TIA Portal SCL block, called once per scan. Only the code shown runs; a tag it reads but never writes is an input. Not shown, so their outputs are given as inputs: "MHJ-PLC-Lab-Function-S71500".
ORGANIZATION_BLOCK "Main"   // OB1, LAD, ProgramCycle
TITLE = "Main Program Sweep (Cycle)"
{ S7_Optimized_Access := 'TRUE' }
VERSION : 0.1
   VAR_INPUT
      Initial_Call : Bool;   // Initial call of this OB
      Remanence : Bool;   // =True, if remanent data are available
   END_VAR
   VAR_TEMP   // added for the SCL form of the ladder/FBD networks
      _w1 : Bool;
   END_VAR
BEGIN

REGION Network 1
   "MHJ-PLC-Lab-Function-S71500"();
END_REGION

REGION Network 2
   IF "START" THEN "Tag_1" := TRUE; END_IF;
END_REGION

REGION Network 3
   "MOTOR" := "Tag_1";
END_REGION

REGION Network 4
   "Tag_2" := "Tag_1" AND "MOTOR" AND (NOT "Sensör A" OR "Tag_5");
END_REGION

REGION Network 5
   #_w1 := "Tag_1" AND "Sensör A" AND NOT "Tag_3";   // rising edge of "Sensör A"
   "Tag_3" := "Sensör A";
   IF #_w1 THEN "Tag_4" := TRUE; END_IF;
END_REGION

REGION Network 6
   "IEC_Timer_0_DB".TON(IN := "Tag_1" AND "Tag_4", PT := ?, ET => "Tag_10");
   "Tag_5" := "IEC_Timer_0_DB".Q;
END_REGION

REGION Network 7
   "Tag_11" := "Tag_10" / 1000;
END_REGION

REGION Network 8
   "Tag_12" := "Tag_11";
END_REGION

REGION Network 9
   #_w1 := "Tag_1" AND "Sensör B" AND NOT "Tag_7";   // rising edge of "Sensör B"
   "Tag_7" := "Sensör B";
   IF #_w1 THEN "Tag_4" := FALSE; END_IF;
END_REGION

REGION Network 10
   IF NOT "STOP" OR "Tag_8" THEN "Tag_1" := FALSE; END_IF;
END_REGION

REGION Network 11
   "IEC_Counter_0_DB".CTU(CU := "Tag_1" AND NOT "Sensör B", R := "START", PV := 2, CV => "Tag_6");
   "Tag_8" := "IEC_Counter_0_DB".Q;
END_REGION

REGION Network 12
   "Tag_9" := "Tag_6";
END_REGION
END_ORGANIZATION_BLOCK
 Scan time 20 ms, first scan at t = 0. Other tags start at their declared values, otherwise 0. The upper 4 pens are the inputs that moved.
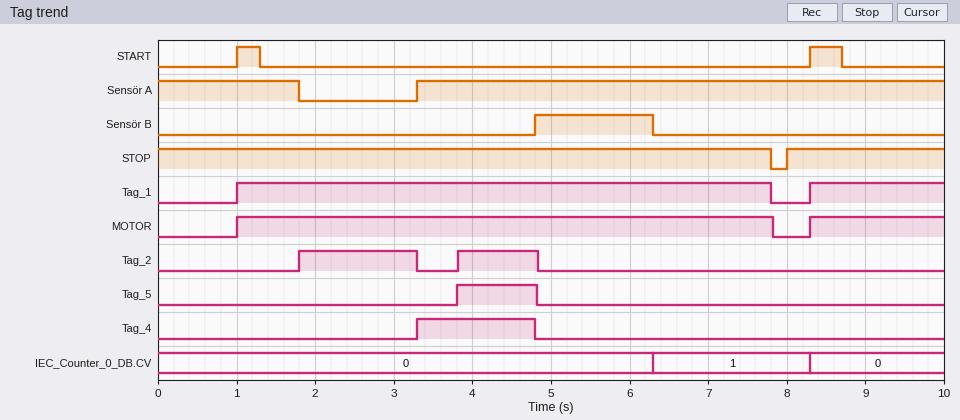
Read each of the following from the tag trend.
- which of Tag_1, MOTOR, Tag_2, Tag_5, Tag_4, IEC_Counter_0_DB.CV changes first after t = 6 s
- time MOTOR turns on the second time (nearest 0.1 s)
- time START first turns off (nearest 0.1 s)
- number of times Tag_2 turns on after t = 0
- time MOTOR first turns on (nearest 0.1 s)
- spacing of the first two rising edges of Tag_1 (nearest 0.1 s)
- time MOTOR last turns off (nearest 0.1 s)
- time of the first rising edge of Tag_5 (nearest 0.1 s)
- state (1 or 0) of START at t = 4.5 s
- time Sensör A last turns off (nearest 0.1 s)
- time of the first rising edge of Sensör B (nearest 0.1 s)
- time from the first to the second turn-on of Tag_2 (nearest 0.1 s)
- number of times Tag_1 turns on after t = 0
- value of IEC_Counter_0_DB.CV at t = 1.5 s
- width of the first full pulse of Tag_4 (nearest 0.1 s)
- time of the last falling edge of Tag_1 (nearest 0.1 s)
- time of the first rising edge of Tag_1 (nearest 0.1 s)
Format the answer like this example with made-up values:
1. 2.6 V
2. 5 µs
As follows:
1. IEC_Counter_0_DB.CV
2. 8.3 s
3. 1.3 s
4. 2
5. 1.0 s
6. 7.3 s
7. 7.8 s
8. 3.8 s
9. 0
10. 1.8 s
11. 4.8 s
12. 2.0 s
13. 2
14. 0
15. 1.5 s
16. 7.8 s
17. 1.0 s
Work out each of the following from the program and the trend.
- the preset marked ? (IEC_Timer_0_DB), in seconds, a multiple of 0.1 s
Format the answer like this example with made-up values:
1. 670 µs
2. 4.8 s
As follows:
1. 0.5 s
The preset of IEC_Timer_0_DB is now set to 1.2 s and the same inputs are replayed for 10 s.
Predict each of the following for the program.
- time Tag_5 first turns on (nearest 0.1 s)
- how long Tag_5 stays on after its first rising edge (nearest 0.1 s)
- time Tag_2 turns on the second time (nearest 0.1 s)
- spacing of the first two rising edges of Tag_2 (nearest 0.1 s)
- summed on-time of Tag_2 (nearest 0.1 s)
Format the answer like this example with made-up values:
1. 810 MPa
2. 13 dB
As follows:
1. 4.5 s
2. 0.3 s
3. 4.5 s
4. 2.7 s
5. 1.8 s
